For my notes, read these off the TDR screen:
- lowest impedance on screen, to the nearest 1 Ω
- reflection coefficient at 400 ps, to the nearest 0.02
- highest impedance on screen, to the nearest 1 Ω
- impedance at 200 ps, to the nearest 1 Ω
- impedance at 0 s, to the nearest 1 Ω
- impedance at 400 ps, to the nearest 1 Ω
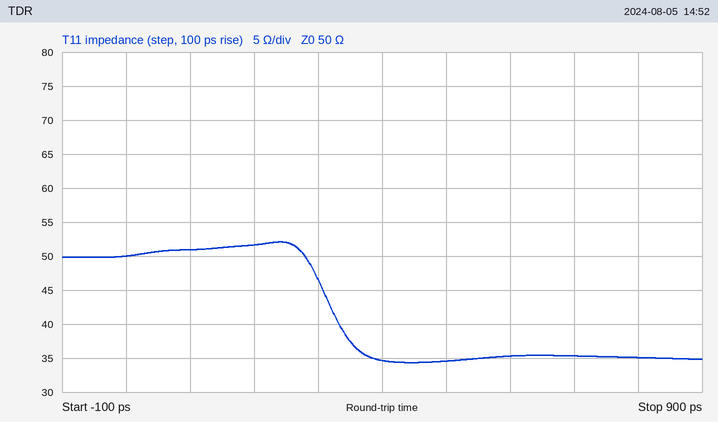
34 Ω
-0.18
52 Ω
52 Ω
50 Ω
35 Ω
